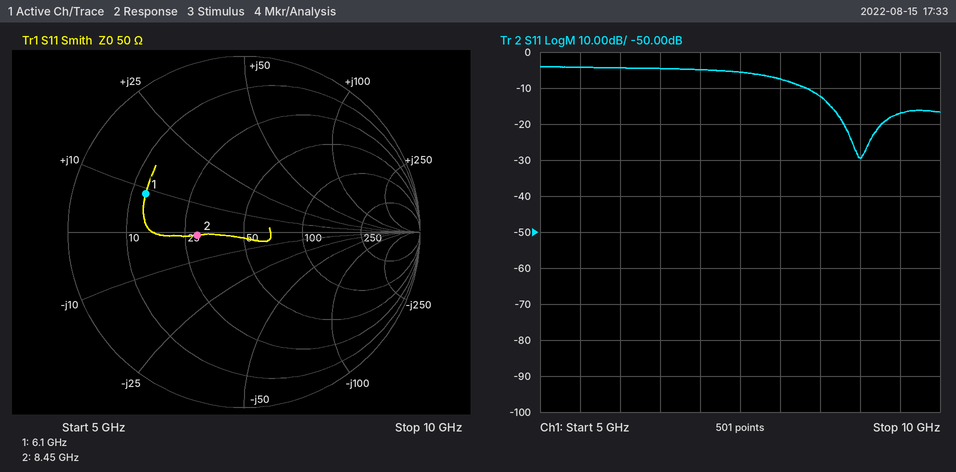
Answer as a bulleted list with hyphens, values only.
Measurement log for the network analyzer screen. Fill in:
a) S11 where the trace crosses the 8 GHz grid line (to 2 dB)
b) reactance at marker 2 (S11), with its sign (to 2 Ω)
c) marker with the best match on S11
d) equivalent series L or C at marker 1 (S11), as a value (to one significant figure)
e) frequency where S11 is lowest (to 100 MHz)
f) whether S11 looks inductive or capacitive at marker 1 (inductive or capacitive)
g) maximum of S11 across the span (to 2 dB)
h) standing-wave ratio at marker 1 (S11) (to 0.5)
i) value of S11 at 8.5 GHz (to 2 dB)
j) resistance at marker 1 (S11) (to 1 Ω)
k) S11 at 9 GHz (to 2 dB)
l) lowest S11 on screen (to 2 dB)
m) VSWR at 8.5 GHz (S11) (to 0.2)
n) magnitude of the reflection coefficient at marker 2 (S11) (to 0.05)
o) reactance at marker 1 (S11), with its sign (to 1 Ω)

- -8 dB
- -2 Ω
- marker 2
- 200 pH
- 9.0 GHz
- inductive
- -4 dB
- 4.0
- -12 dB
- 13 Ω
- -30 dB
- -30 dB
- 1.6
- 0.25
- +9 Ω
